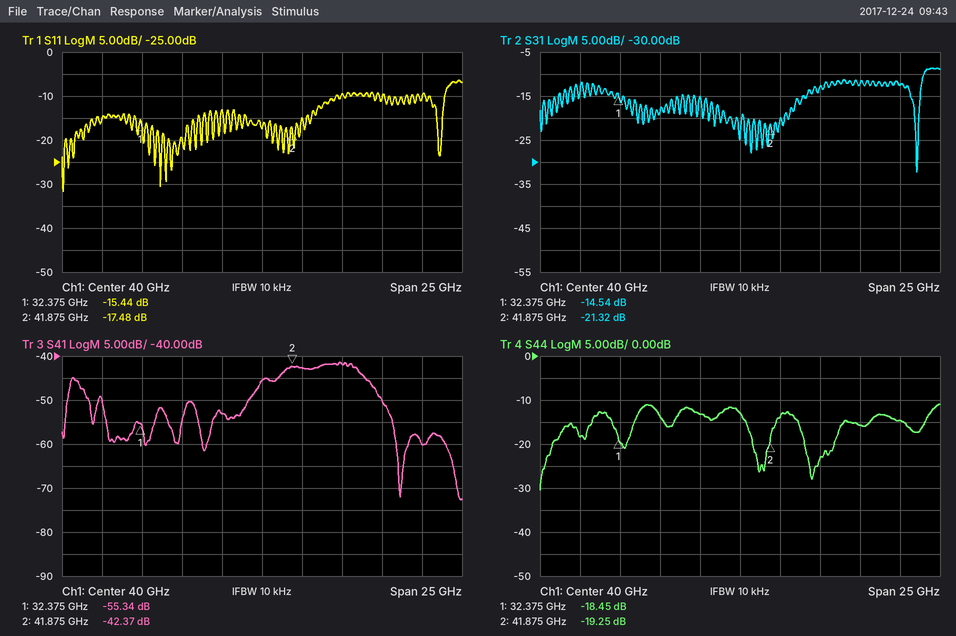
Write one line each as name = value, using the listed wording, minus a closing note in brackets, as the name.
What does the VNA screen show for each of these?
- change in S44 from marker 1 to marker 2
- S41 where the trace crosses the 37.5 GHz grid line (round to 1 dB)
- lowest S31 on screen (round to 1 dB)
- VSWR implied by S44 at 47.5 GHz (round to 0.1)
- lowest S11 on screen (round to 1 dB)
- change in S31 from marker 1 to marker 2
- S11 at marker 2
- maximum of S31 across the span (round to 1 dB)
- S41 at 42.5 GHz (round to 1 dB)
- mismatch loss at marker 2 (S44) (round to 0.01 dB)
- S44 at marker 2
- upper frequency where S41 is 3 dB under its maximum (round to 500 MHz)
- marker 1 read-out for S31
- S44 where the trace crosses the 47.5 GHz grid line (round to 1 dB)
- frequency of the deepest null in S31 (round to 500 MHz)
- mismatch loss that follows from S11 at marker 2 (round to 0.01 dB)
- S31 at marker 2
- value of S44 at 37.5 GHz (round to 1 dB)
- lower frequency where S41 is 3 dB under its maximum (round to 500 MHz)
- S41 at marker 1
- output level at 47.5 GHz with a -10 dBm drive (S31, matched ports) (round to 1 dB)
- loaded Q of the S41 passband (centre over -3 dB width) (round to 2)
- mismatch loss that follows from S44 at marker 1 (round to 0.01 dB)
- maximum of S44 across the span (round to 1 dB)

change in S44 from marker 1 to marker 2 = -0.80 dB
S41 where the trace crosses the 37.5 GHz grid line = -53 dB
lowest S31 on screen = -32 dB
VSWR implied by S44 at 47.5 GHz = 1.4
lowest S11 on screen = -32 dB
change in S31 from marker 1 to marker 2 = -6.78 dB
S11 at marker 2 = -17.48 dB
maximum of S31 across the span = -9 dB
S41 at 42.5 GHz = -43 dB
mismatch loss at marker 2 (S44) = 0.05 dB
S44 at marker 2 = -19.25 dB
upper frequency where S41 is 3 dB under its maximum = 46.5 GHz
marker 1 read-out for S31 = -14.54 dB
S44 where the trace crosses the 47.5 GHz grid line = -16 dB
frequency of the deepest null in S31 = 51.0 GHz
mismatch loss that follows from S11 at marker 2 = 0.08 dB
S31 at marker 2 = -21.32 dB
value of S44 at 37.5 GHz = -13 dB
lower frequency where S41 is 3 dB under its maximum = 41.0 GHz
S41 at marker 1 = -55.34 dB
output level at 47.5 GHz with a -10 dBm drive (S31, matched ports) = -22 dBm
loaded Q of the S41 passband (centre over -3 dB width) = 8
mismatch loss that follows from S44 at marker 1 = 0.06 dB
maximum of S44 across the span = -11 dB
